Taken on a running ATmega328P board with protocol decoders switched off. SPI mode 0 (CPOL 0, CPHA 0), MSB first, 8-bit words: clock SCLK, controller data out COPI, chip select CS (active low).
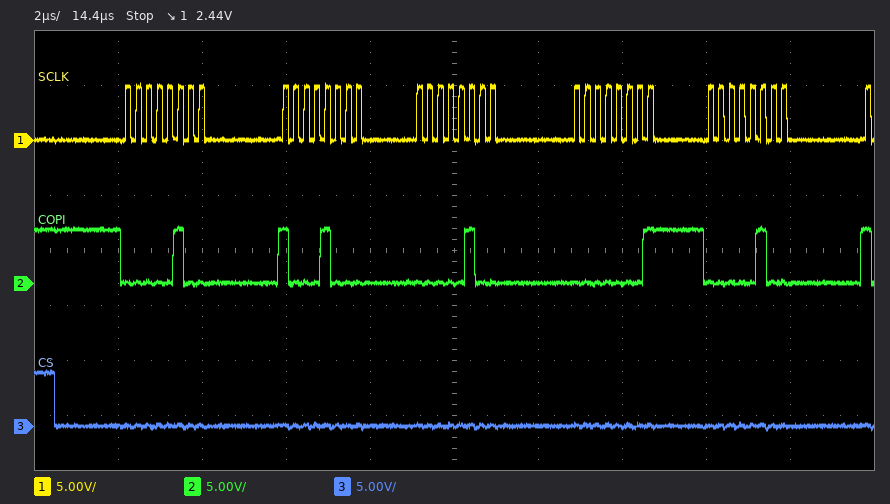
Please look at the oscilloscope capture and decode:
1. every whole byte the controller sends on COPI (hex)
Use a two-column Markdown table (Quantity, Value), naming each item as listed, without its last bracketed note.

| Quantity | Value |
|---|---|
| every whole byte the controller sends on COPI | 04 88 04 01 04 |
